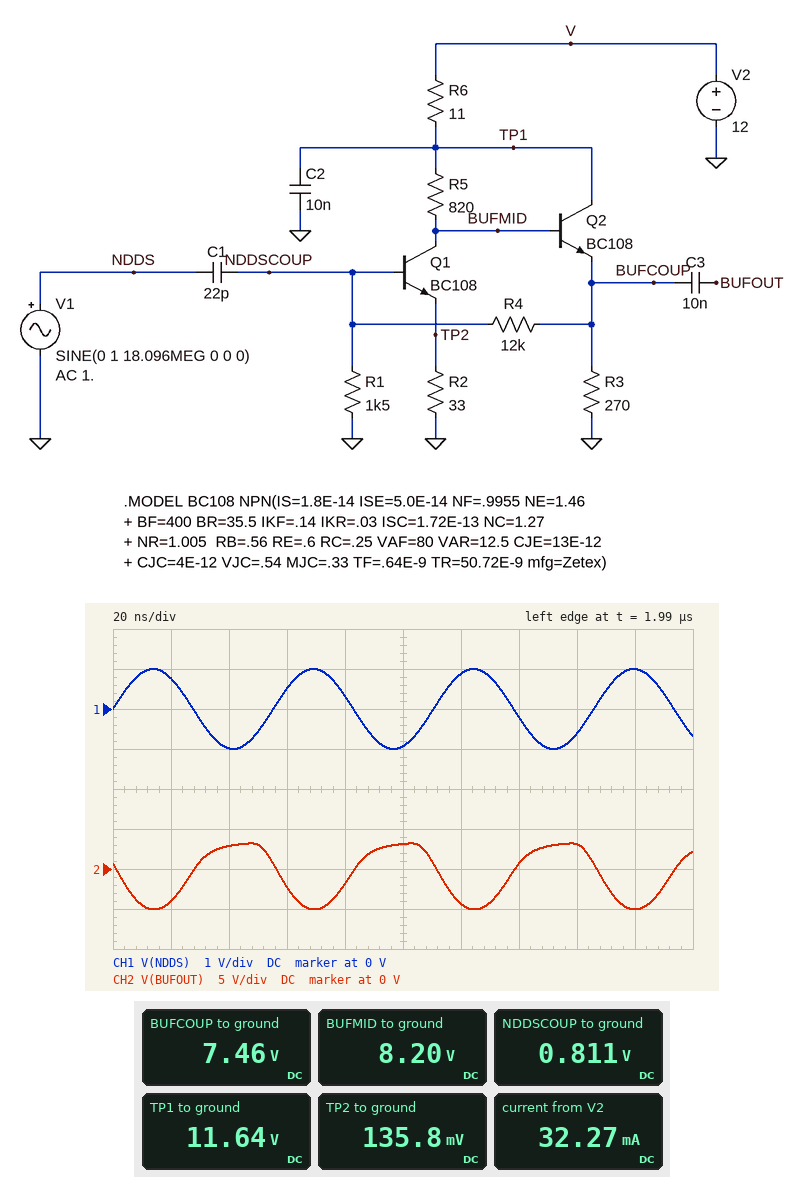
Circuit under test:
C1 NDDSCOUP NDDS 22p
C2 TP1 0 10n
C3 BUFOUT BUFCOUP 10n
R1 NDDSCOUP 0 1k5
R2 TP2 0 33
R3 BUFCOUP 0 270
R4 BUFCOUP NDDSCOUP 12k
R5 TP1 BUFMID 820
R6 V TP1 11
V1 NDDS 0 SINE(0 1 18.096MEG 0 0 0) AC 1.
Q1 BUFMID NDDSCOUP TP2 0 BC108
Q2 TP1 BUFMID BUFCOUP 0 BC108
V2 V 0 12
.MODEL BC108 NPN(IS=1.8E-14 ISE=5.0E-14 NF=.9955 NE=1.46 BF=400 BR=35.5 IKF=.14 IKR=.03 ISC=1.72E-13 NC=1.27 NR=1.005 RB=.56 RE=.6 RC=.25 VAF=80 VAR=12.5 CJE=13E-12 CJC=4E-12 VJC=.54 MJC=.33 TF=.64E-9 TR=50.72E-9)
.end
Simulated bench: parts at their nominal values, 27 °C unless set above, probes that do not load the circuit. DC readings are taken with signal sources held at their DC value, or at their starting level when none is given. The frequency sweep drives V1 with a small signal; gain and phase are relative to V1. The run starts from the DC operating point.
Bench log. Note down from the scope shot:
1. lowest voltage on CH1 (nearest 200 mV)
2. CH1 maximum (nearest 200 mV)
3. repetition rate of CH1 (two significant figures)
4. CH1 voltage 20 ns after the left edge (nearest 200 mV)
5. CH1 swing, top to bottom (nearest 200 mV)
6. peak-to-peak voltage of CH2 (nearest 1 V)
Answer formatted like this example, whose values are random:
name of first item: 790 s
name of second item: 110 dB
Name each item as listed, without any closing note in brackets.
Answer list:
lowest voltage on CH1: -1.0 V
CH1 maximum: 1.0 V
repetition rate of CH1: 18 MHz
CH1 voltage 20 ns after the left edge: 800 mV
CH1 swing, top to bottom: 2.0 V
peak-to-peak voltage of CH2: 8 V
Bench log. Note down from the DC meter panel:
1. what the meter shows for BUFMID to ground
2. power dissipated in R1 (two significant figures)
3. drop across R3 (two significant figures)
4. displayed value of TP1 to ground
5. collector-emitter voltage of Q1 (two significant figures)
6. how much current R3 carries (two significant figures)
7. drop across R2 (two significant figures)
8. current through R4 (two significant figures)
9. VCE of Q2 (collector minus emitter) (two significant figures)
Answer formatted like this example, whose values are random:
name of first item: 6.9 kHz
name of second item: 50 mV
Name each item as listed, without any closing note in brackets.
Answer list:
what the meter shows for BUFMID to ground: 8.20 V
power dissipated in R1: 440 µW
drop across R3: 7.5 V
displayed value of TP1 to ground: 11.64 V
collector-emitter voltage of Q1: 8.1 V
how much current R3 carries: 28 mA
drop across R2: 140 mV
current through R4: 550 µA
VCE of Q2 (collector minus emitter): 4.2 V
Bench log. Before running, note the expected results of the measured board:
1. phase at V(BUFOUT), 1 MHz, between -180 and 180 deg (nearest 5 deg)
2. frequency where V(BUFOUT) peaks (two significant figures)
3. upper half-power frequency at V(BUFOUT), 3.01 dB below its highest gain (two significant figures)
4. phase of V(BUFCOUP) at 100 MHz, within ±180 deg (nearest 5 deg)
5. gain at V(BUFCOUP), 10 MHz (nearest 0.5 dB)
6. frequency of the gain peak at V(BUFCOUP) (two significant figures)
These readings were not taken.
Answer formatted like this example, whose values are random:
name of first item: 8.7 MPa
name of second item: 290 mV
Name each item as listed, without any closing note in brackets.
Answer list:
phase at V(BUFOUT), 1 MHz, between -180 and 180 deg: -100 deg
frequency where V(BUFOUT) peaks: 17 MHz
upper half-power frequency at V(BUFOUT), 3.01 dB below its highest gain: 64 MHz
phase of V(BUFCOUP) at 100 MHz, within ±180 deg: 115 deg
gain at V(BUFCOUP), 10 MHz: 14.5 dB
frequency of the gain peak at V(BUFCOUP): 17 MHz
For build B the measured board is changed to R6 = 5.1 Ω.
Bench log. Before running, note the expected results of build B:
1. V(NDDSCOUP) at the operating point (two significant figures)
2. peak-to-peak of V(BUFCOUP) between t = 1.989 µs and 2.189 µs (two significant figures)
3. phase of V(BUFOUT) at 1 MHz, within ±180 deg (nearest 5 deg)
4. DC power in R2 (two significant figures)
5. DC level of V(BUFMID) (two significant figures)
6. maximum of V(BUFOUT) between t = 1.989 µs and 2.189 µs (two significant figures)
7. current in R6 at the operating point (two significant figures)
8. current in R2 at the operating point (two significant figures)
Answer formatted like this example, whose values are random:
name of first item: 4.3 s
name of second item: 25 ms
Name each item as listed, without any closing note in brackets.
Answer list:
V(NDDSCOUP) at the operating point: 820 mV
peak-to-peak of V(BUFCOUP) between t = 1.989 µs and 2.189 µs: 8.4 V
phase of V(BUFOUT) at 1 MHz, within ±180 deg: -100 deg
DC power in R2: 600 µW
DC level of V(BUFMID): 8.3 V
maximum of V(BUFOUT) between t = 1.989 µs and 2.189 µs: 3.3 V
current in R6 at the operating point: 33 mA
current in R2 at the operating point: 4.3 mA
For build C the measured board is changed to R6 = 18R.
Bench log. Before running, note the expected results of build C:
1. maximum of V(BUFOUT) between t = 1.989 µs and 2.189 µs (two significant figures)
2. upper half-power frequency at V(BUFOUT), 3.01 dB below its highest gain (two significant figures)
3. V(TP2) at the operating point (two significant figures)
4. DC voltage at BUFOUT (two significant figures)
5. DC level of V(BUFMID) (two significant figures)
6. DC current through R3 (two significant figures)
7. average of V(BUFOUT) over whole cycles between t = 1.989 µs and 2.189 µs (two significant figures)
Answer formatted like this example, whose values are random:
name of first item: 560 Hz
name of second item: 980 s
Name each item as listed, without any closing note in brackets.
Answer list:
maximum of V(BUFOUT) between t = 1.989 µs and 2.189 µs: 3.1 V
upper half-power frequency at V(BUFOUT), 3.01 dB below its highest gain: 63 MHz
V(TP2) at the operating point: 130 mV
DC voltage at BUFOUT: 7.4 V
DC level of V(BUFMID): 8.1 V
DC current through R3: 27 mA
average of V(BUFOUT) over whole cycles between t = 1.989 µs and 2.189 µs: -440 mV
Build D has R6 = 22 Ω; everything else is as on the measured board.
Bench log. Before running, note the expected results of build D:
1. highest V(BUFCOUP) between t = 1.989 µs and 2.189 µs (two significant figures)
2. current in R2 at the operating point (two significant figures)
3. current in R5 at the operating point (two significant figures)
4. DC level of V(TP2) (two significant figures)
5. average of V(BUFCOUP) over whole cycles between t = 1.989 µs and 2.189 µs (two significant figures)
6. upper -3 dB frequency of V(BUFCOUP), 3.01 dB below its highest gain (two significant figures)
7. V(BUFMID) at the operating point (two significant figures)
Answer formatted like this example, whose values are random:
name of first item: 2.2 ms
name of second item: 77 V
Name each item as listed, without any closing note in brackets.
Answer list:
highest V(BUFCOUP) between t = 1.989 µs and 2.189 µs: 10 V
current in R2 at the operating point: 3.8 mA
current in R5 at the operating point: 3.9 mA
DC level of V(TP2): 130 mV
average of V(BUFCOUP) over whole cycles between t = 1.989 µs and 2.189 µs: 6.9 V
upper -3 dB frequency of V(BUFCOUP), 3.01 dB below its highest gain: 63 MHz
V(BUFMID) at the operating point: 8.1 V
